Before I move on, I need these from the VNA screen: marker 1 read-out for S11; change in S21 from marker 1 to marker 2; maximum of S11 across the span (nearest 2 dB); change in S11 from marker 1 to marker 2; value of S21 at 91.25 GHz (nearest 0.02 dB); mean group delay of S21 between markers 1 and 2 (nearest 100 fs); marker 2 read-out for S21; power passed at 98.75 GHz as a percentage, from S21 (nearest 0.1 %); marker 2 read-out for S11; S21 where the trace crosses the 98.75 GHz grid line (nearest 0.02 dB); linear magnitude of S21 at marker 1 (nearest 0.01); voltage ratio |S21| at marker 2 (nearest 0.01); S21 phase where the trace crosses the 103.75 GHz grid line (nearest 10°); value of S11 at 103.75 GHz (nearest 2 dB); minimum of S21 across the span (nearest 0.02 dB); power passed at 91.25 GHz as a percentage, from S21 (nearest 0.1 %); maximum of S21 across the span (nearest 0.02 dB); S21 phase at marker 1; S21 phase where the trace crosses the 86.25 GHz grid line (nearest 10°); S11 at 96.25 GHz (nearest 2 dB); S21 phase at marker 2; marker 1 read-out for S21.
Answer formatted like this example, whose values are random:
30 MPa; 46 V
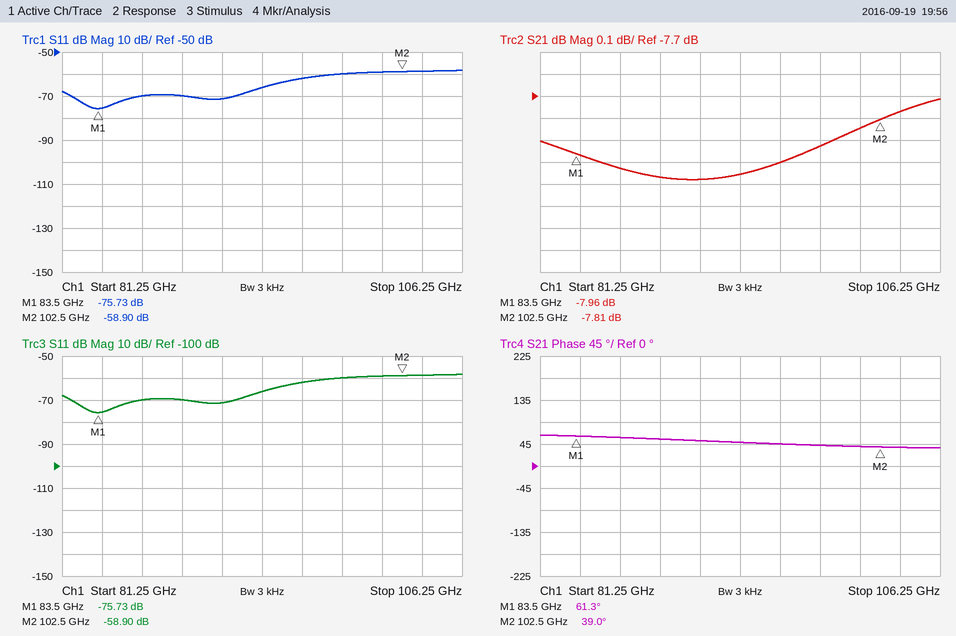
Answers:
-75.73 dB; 0.15 dB; -58 dB; 16.83 dB; -8.08 dB; 3.3 ps; -7.81 dB; 16.1 %; -58.90 dB; -7.92 dB; 0.40; 0.41; 40°; -58 dB; -8.08 dB; 15.6 %; -7.72 dB; 61.3°; 60°; -62 dB; 39.0°; -7.96 dB
